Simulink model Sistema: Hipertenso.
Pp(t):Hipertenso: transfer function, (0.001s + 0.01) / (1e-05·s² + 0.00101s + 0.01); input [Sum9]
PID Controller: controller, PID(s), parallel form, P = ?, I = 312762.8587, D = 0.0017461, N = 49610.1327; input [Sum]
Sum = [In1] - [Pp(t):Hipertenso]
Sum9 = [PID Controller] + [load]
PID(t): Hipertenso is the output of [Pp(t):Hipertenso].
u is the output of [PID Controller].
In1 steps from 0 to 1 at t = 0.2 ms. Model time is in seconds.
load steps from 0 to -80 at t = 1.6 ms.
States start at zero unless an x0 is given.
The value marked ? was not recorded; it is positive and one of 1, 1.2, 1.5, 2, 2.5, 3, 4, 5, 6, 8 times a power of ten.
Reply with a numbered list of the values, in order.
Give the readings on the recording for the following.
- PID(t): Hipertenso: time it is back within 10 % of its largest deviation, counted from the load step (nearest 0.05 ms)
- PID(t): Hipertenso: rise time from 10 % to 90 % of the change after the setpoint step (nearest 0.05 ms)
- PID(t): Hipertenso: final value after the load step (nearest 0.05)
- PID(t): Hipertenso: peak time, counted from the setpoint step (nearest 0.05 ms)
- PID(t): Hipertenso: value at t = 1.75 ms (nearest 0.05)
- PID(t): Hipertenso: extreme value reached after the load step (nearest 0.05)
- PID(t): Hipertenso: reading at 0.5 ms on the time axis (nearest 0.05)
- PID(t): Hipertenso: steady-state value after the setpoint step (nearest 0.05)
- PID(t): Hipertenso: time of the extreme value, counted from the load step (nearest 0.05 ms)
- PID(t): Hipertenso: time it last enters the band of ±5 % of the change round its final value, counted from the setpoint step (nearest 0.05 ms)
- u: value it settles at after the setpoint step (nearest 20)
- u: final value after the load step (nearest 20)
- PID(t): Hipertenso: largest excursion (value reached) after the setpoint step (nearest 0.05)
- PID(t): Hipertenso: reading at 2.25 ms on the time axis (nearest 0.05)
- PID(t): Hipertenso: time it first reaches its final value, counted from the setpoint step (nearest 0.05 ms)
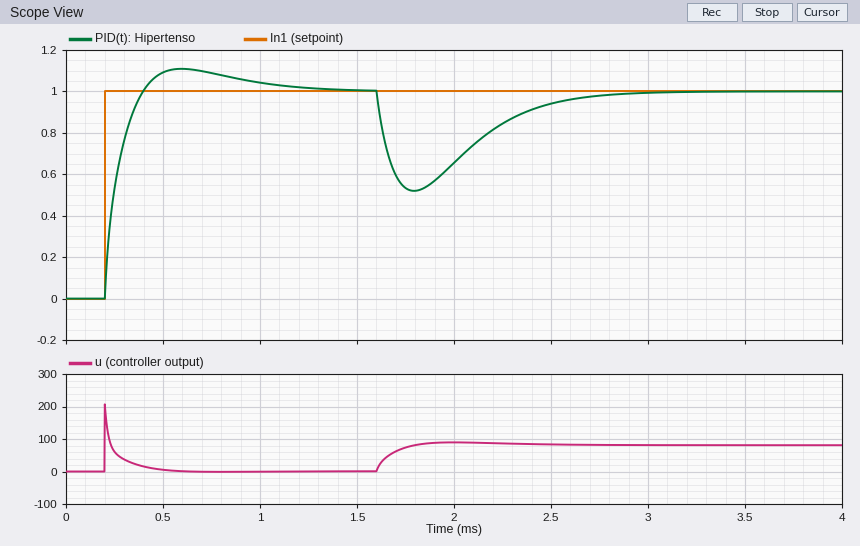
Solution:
1. 0.95 ms
2. 0.15 ms
3. 1.00
4. 0.40 ms
5. 0.55
6. 0.50
7. 1.10
8. 1.00
9. 0.20 ms
10. 0.75 ms
11. 0
12. 80
13. 1.10
14. 0.85
15. 0.20 ms
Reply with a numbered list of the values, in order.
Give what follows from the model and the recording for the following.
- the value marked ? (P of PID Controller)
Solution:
1. 120
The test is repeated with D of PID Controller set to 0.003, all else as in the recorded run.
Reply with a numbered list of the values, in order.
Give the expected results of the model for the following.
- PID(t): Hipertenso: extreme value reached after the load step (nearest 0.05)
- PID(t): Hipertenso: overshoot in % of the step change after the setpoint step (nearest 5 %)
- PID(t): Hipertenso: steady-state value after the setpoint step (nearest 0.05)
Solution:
1. 0.55
2. 10 %
3. 1.00
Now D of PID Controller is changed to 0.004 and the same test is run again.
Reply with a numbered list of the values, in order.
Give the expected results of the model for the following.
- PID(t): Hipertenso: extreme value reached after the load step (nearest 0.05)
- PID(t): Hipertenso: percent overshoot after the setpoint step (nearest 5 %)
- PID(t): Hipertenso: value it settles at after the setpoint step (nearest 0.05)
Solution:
1. 0.55
2. 10 %
3. 1.00
